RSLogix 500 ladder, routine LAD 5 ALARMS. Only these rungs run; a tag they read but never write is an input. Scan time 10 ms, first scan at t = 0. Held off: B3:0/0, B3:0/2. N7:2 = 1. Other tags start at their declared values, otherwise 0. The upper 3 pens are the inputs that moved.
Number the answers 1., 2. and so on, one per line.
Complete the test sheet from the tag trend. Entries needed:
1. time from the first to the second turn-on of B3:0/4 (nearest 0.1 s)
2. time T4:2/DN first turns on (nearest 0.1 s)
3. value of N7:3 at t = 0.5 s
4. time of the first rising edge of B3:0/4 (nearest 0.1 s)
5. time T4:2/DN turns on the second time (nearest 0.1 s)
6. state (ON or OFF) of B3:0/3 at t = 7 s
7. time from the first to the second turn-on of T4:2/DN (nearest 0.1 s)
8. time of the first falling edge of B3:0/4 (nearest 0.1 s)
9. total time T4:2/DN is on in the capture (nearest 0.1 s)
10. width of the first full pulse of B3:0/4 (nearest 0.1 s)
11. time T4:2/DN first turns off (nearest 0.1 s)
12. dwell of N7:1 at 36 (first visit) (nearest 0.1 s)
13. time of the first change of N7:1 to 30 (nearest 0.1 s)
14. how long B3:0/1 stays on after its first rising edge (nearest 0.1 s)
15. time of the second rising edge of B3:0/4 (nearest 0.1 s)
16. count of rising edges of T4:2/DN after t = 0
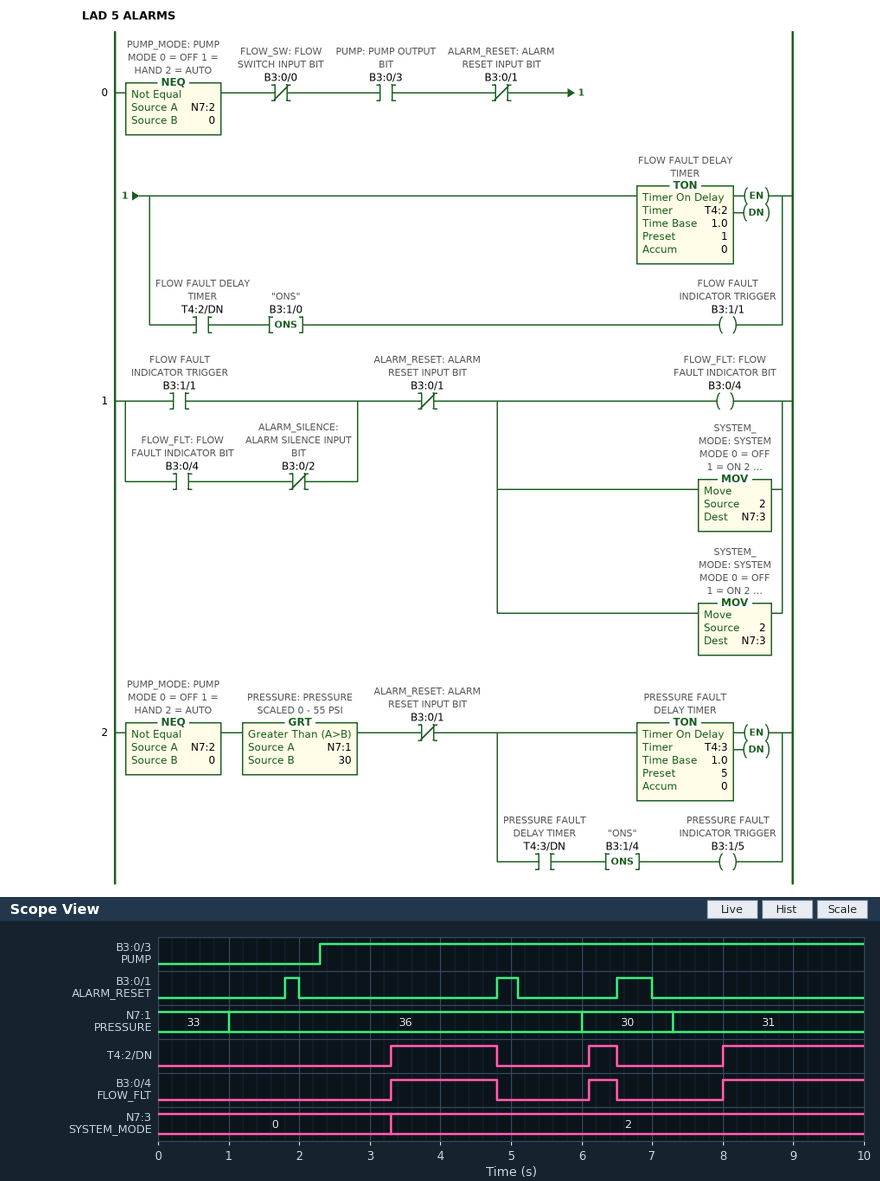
1. 2.8 s
2. 3.3 s
3. 0
4. 3.3 s
5. 6.1 s
6. ON
7. 2.8 s
8. 4.8 s
9. 3.9 s
10. 1.5 s
11. 4.8 s
12. 5.0 s
13. 6.0 s
14. 0.2 s
15. 6.1 s
16. 3
